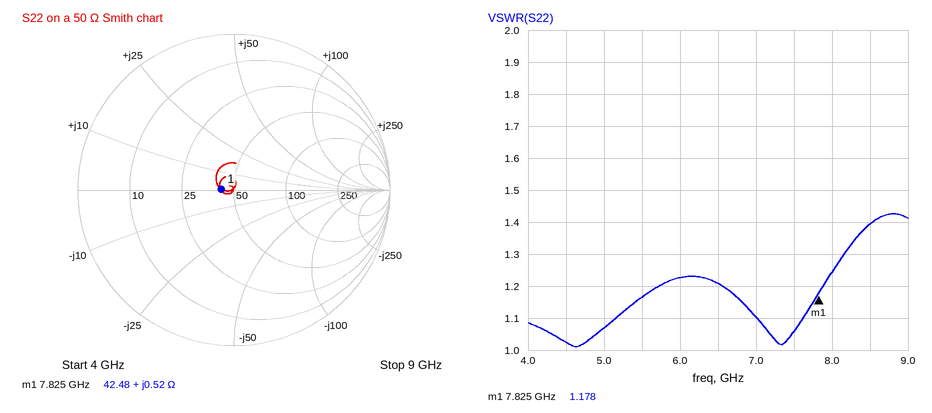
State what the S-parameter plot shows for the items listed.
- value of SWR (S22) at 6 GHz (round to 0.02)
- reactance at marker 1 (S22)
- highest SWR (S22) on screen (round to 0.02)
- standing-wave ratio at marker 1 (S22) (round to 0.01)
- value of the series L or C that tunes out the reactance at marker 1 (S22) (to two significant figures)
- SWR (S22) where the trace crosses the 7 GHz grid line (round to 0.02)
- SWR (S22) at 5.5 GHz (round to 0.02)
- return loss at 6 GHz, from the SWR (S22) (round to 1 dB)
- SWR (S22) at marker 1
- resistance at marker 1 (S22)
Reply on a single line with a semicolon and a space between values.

1.22; +0.52 Ω; 1.42; 1.18; 39 pF; 1.10; 1.16; 20 dB; 1.178; 42.48 Ω
